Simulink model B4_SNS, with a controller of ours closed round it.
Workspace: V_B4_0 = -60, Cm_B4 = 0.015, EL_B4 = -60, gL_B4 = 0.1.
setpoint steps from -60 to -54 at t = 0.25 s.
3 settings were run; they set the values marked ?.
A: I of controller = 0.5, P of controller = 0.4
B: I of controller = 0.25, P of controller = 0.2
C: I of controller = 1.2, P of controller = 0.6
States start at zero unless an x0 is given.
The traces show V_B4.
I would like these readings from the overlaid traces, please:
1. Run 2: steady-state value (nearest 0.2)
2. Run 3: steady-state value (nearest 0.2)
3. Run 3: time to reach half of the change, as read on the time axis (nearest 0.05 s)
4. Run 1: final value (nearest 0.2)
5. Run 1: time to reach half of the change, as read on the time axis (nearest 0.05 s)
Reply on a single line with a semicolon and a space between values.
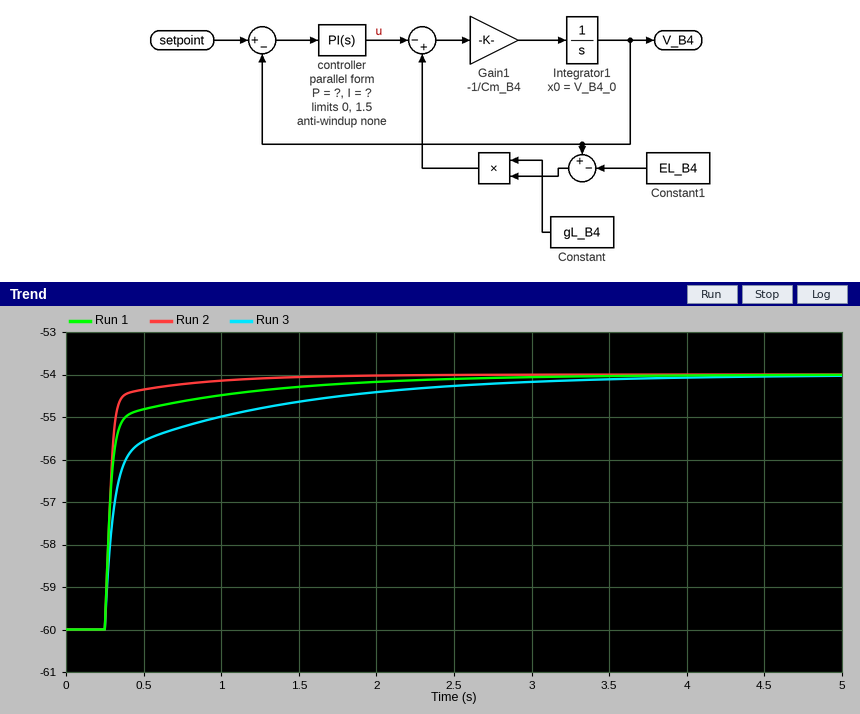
-54.0; -54.0; 0.30 s; -54.0; 0.30 s
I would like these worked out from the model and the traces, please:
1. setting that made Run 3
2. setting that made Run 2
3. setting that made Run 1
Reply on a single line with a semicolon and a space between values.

B; C; A
